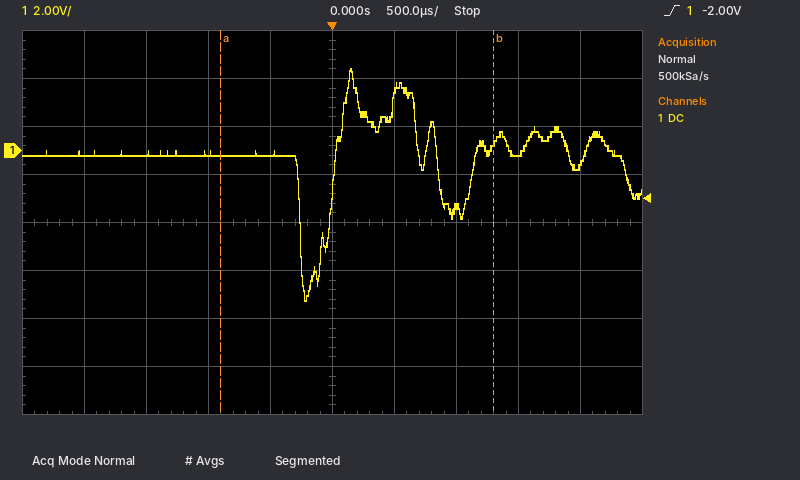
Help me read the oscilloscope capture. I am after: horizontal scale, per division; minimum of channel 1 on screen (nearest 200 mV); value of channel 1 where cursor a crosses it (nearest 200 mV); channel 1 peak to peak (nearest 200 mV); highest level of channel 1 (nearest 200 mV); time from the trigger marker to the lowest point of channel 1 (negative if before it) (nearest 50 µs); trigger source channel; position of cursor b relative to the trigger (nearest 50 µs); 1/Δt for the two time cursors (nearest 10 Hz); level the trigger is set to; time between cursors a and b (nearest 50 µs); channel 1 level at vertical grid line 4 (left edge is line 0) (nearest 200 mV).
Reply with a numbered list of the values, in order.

1. 500 µs
2. -6.2 V
3. -200 mV
4. 9.6 V
5. 3.4 V
6. -200 µs
7. channel 1
8. +1.30 ms
9. 450 Hz
10. -2.00 V
11. 2.20 ms
12. -200 mV
